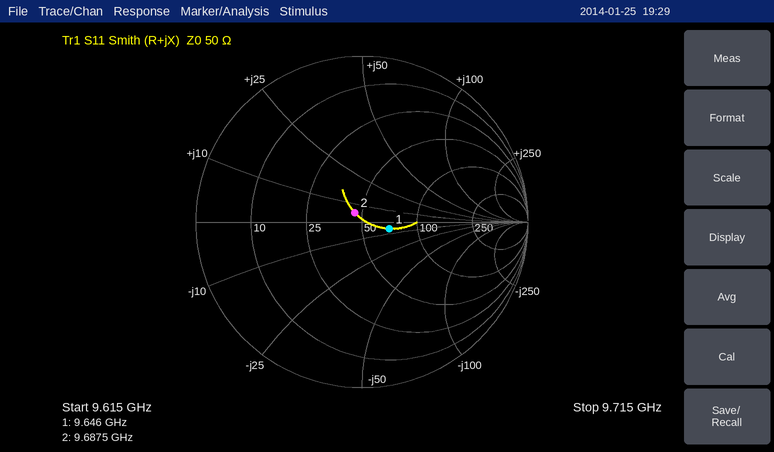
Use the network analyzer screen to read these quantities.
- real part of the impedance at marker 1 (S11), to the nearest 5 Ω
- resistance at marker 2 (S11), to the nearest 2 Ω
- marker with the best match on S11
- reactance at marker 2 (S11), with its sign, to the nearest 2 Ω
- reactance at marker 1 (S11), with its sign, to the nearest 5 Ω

70 Ω
46 Ω
marker 2
+6 Ω
-5 Ω
